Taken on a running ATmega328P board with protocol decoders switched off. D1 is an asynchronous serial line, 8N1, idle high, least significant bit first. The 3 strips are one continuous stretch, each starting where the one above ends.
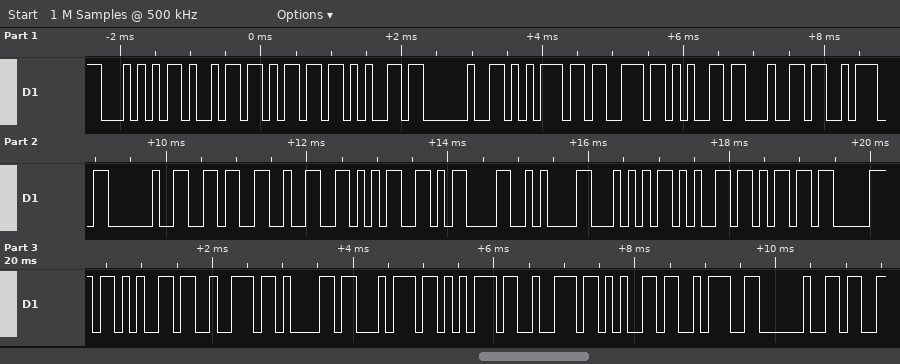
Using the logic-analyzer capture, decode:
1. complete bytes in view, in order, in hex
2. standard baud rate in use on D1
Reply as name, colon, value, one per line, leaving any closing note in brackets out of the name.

complete bytes in view, in order, in hex: 0x54 0x69 0x6D 0x65 0x20 0x75 0x73 0x65 0x64 0x3A 0x20 0x36 0x32 0x35 0x0D 0x0A 0x54 0x65 0x6D 0x70 0x65 0x72 0x61 0x74 0x75 0x72 0x65 0x3A 0x20
standard baud rate in use on D1: 9600 baud
